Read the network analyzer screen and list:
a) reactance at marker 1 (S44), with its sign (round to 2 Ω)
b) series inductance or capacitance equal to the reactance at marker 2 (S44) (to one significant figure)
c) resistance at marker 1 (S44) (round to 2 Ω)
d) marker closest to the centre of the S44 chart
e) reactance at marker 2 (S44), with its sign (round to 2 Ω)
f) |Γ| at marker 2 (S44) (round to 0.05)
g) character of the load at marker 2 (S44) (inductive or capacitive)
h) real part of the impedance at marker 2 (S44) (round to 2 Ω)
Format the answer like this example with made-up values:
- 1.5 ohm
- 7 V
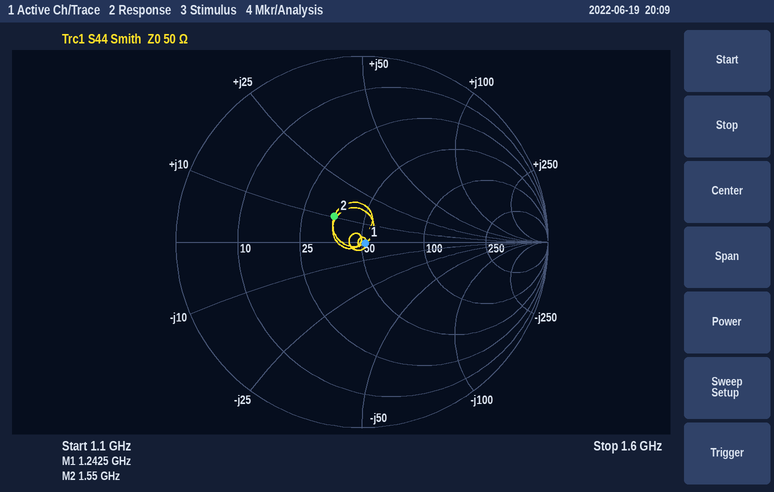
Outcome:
- 0 Ω
- 1 nH
- 52 Ω
- marker 1
- +10 Ω
- 0.20
- inductive
- 36 Ω
